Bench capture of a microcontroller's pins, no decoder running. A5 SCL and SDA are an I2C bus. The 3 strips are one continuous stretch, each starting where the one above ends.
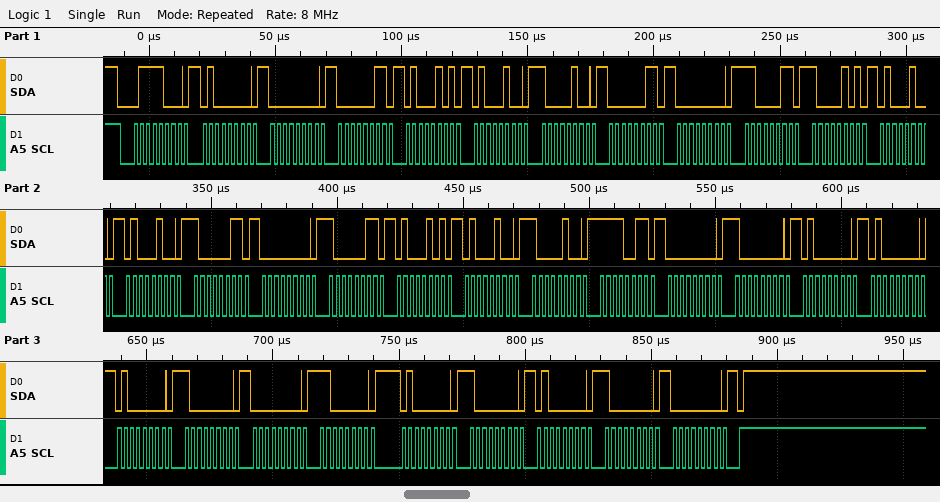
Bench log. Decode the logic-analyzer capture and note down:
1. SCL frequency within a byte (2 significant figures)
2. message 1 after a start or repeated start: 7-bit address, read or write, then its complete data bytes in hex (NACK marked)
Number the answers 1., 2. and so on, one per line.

1. 400 kHz
2. 0x3C write: 40 00 03 45 44 84 03 00 C3 85 44 44 83 00 83 45 44 84 F3 00 80 40 40 40 80 00 C0 40 80 40 80 00
